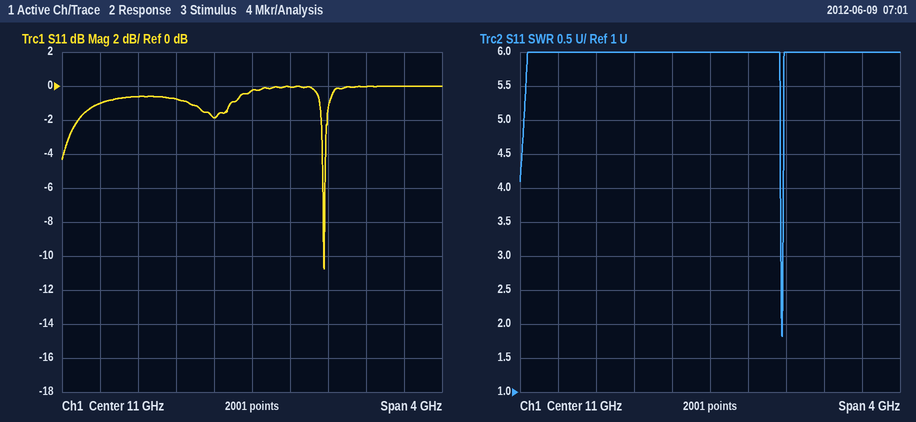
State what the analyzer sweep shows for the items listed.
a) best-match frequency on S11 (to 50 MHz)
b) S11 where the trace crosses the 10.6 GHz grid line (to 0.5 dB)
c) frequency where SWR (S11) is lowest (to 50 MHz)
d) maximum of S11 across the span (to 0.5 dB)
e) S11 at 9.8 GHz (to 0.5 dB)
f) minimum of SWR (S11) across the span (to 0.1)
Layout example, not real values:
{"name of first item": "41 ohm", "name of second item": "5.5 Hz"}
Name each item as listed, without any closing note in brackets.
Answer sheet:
{"best-match frequency on S11": "11.75 GHz", "S11 where the trace crosses the 10.6 GHz grid line": "-2.0 dB", "frequency where SWR (S11) is lowest": "11.75 GHz", "maximum of S11 across the span": "0.0 dB", "S11 at 9.8 GHz": "-0.5 dB", "minimum of SWR (S11) across the span": "1.8"}
